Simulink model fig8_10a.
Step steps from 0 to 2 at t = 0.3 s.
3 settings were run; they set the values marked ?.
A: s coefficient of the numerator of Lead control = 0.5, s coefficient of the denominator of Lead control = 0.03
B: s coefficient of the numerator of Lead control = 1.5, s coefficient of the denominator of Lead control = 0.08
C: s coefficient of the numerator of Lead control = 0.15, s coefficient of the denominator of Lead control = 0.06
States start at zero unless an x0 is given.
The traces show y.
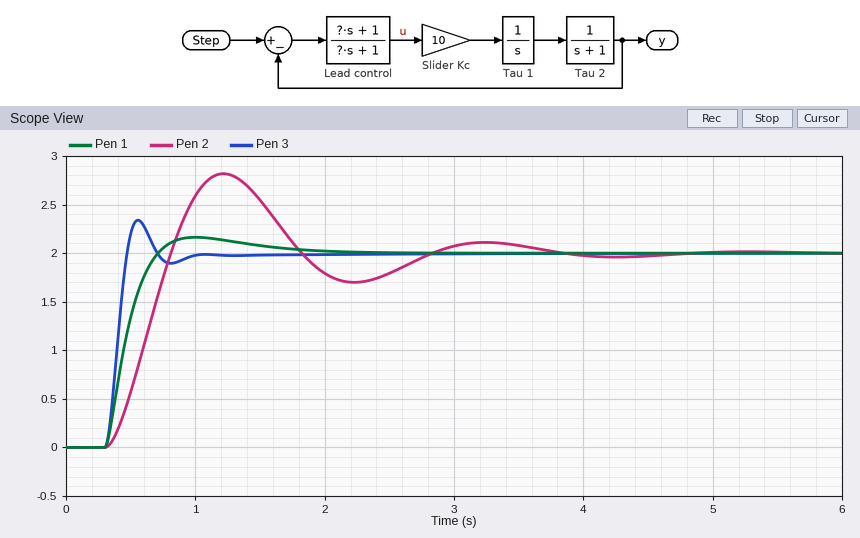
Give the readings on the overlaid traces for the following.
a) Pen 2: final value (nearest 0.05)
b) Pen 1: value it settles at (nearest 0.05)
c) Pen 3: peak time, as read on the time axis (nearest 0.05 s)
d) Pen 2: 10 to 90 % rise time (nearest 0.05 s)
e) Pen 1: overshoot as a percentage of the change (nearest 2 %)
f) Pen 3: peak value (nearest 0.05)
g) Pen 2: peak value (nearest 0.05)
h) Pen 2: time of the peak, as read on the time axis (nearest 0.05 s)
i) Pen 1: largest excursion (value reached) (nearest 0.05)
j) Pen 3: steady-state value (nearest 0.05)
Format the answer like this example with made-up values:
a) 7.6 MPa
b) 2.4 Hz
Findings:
a) 2.00
b) 2.00
c) 0.55 s
d) 0.35 s
e) 8 %
f) 2.35
g) 2.80
h) 1.20 s
i) 2.15
j) 2.00
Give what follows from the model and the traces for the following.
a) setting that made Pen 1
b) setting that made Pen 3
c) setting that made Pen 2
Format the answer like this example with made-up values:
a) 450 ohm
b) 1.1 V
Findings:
a) A
b) B
c) C
